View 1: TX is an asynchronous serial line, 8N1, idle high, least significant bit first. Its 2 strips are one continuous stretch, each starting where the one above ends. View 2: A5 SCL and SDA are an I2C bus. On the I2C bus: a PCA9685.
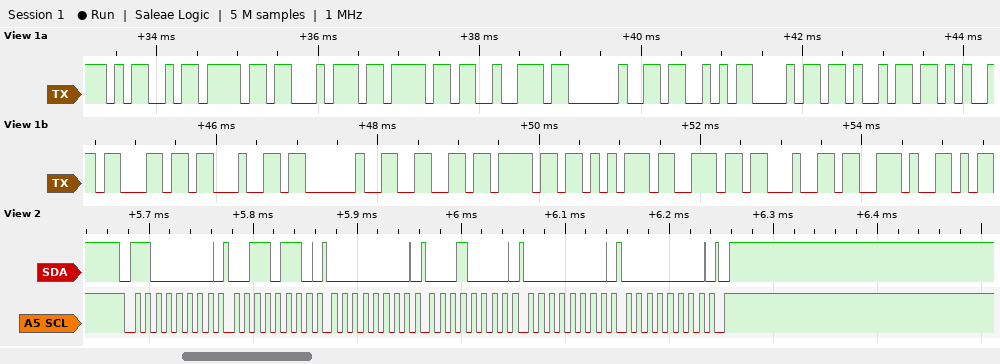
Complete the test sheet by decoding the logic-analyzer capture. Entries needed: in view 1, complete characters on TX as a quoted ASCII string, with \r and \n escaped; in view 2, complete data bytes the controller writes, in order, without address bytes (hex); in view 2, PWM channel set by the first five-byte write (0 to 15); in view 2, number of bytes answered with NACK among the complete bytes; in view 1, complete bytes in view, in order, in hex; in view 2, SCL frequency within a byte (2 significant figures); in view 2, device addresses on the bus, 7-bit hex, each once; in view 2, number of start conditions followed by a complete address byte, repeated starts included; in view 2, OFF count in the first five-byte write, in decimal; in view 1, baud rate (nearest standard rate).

"Motor Shield found."
36 00 10 00 00
12
0
0x4D 0x6F 0x74 0x6F 0x72 0x20 0x53 0x68 0x69 0x65 0x6C 0x64 0x20 0x66 0x6F 0x75 0x6E 0x64 0x2E
100 kHz
0x60
1
0
9600 baud
